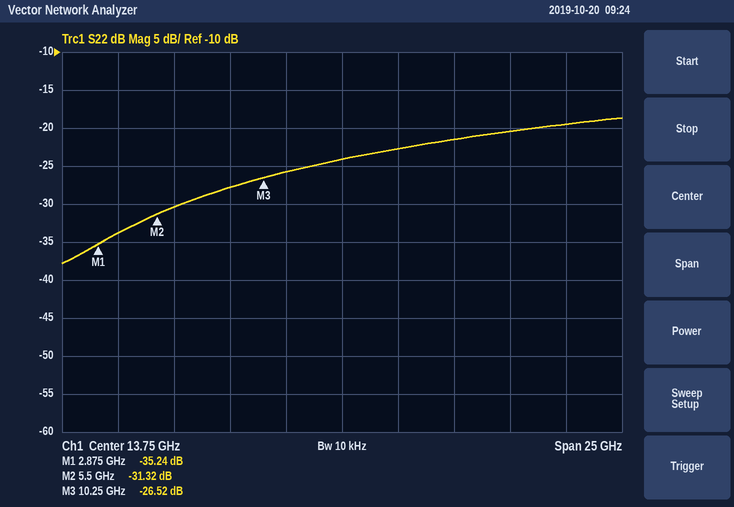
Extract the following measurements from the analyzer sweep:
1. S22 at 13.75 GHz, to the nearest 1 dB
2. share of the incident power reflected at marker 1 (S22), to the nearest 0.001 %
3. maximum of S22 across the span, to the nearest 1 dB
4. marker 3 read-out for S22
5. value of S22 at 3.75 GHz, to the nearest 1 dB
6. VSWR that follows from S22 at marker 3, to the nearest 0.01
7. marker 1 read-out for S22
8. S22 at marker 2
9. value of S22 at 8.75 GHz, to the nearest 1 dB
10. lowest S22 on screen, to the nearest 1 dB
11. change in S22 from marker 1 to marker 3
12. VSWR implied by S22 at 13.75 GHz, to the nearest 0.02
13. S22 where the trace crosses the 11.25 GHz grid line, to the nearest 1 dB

-24 dB
0.030 %
-19 dB
-26.52 dB
-34 dB
1.10
-35.24 dB
-31.32 dB
-28 dB
-38 dB
8.72 dB
1.14
-26 dB
